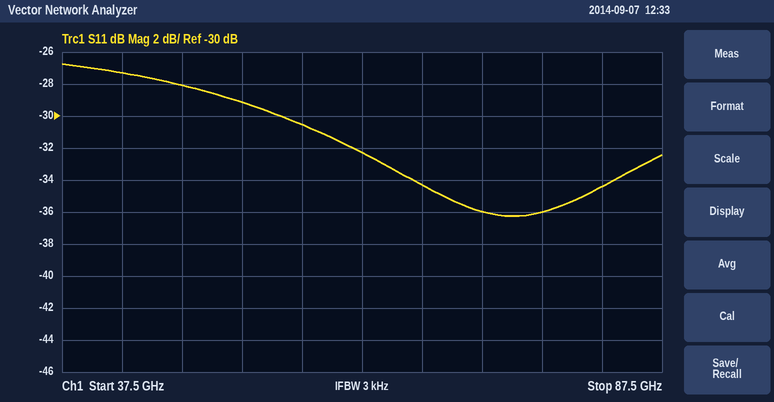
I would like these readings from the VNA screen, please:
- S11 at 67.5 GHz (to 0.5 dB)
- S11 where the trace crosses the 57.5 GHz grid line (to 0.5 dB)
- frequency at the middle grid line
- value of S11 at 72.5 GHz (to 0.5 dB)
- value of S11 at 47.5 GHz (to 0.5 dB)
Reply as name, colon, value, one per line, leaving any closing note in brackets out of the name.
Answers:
S11 at 67.5 GHz: -34.5 dB
S11 where the trace crosses the 57.5 GHz grid line: -30.5 dB
frequency at the middle grid line: 62.5 GHz
value of S11 at 72.5 GHz: -36.0 dB
value of S11 at 47.5 GHz: -28.0 dB
